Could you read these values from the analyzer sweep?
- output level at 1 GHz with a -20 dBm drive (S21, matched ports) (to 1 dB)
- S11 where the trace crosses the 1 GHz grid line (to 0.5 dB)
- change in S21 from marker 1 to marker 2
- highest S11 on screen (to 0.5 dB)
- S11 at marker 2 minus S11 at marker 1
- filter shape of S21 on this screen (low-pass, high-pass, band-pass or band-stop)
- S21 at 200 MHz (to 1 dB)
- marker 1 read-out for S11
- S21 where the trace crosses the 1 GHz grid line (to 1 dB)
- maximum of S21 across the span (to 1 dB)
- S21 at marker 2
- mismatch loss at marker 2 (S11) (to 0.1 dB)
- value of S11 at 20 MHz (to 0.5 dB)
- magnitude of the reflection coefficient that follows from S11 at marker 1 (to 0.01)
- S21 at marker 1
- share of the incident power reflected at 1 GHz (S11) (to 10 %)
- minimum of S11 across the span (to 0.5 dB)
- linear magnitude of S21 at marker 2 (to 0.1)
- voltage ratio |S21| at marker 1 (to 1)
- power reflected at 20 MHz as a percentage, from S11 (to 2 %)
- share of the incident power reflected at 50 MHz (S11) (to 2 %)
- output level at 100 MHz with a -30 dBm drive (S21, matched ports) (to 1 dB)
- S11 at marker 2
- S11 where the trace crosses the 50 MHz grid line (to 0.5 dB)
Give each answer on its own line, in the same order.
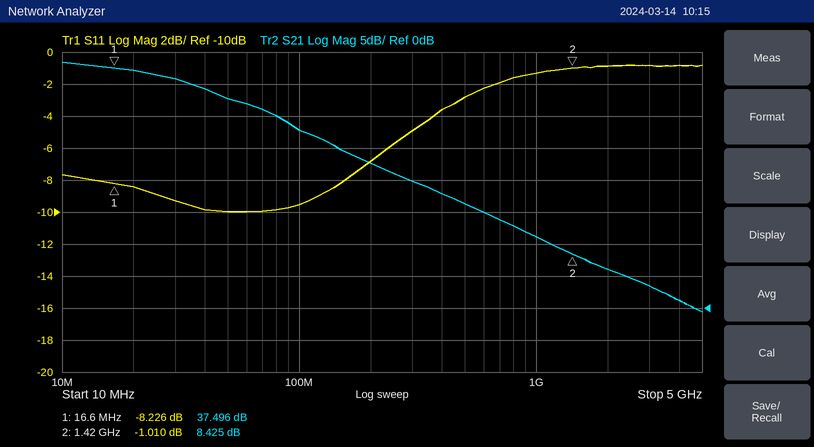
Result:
-9 dBm
-1.5 dB
-29.071 dB
-1.0 dB
7.216 dB
low-pass
23 dB
-8.226 dB
11 dB
38 dB
8.425 dB
6.8 dB
-8.5 dB
0.39
37.496 dB
70 %
-10.0 dB
2.6
75
14 %
10 %
-2 dBm
-1.010 dB
-10.0 dB
